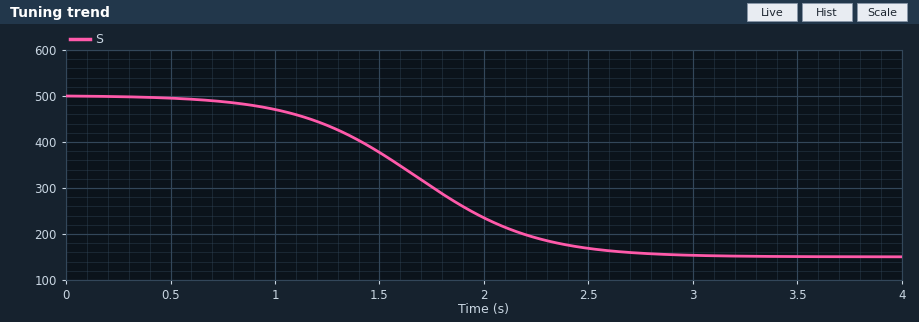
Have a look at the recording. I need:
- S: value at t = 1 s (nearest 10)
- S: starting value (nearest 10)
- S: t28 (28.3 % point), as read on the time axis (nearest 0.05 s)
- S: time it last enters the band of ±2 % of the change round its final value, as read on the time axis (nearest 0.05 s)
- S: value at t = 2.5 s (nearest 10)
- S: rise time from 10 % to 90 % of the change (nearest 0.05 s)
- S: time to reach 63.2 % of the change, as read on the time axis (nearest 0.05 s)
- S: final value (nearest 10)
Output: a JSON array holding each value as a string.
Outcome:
["470", "500", "1.40 s", "2.80 s", "170", "1.25 s", "1.85 s", "150"]
